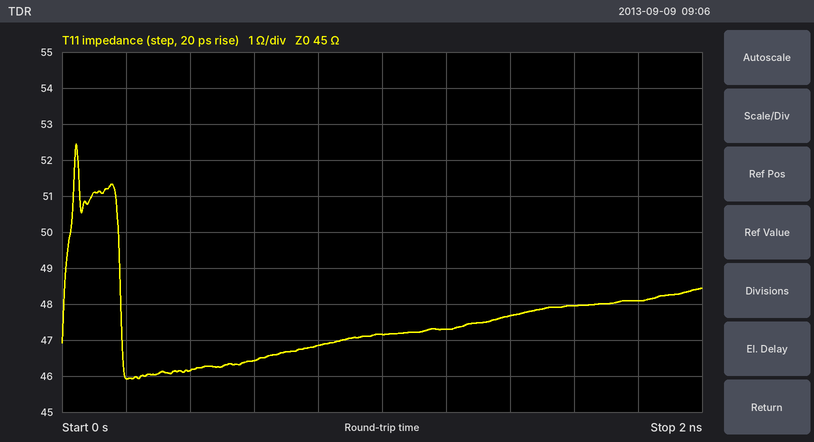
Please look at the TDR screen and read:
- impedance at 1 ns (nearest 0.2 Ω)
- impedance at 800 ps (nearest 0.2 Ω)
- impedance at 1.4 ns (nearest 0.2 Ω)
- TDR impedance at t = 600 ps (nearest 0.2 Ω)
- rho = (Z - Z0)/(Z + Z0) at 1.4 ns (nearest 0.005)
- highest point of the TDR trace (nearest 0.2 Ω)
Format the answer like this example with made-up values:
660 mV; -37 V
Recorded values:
47.2 Ω; 46.8 Ω; 47.6 Ω; 46.4 Ω; +0.030; 52.4 Ω
